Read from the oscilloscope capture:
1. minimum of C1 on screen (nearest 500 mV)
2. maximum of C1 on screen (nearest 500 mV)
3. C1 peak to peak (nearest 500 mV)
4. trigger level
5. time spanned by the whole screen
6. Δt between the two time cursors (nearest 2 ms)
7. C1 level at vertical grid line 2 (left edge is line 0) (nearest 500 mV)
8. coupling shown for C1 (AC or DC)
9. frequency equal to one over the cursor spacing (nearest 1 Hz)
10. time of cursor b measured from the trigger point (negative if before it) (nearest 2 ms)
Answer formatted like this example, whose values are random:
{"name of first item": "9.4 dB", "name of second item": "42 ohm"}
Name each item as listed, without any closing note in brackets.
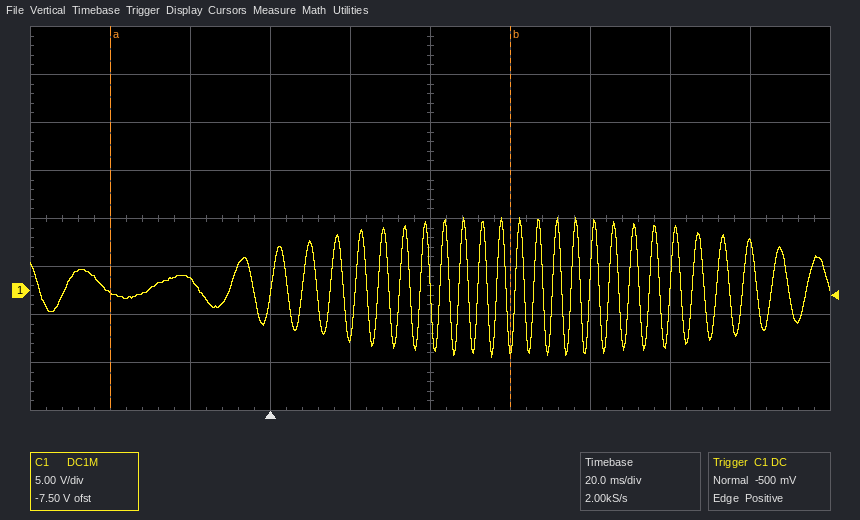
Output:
{"minimum of C1 on screen": "-7.0 V", "maximum of C1 on screen": "7.5 V", "C1 peak to peak": "14.5 V", "trigger level": "-500 mV", "time spanned by the whole screen": "200 ms", "Δt between the two time cursors": "100 ms", "C1 level at vertical grid line 2 (left edge is line 0)": "1.0 V", "coupling shown for C1": "DC", "frequency equal to one over the cursor spacing": "10 Hz", "time of cursor b measured from the trigger point (negative if before it)": "+60 ms"}
